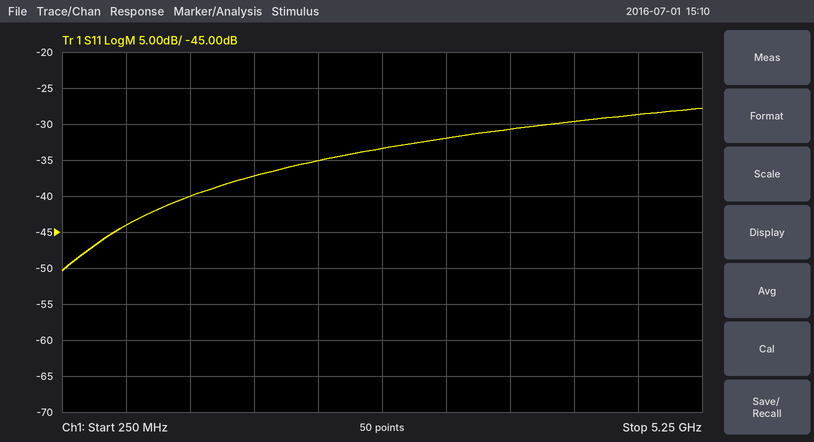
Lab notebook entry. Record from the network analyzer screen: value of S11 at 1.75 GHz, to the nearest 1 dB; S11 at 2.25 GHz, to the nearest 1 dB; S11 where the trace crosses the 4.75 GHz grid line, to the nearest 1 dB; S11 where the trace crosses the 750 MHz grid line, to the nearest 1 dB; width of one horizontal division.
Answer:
-37 dB
-35 dB
-29 dB
-44 dB
500 MHz
